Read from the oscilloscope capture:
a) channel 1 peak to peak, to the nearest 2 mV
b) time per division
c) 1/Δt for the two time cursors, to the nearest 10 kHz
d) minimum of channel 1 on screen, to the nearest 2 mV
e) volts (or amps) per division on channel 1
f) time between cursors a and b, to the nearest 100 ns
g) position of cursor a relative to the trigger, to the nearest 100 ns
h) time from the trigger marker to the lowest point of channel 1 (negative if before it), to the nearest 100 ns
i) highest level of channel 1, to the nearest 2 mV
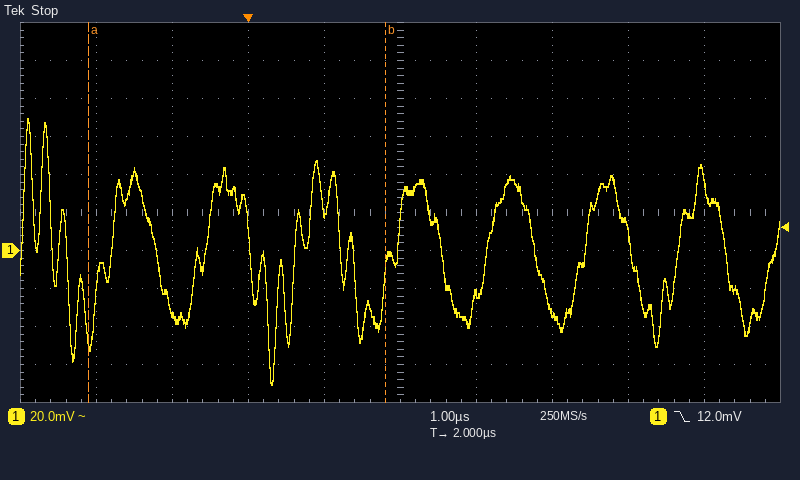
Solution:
140 mV
1 µs
260 kHz
-70 mV
20 mV
3.9 µs
-2.1 µs
+300 ns
70 mV
